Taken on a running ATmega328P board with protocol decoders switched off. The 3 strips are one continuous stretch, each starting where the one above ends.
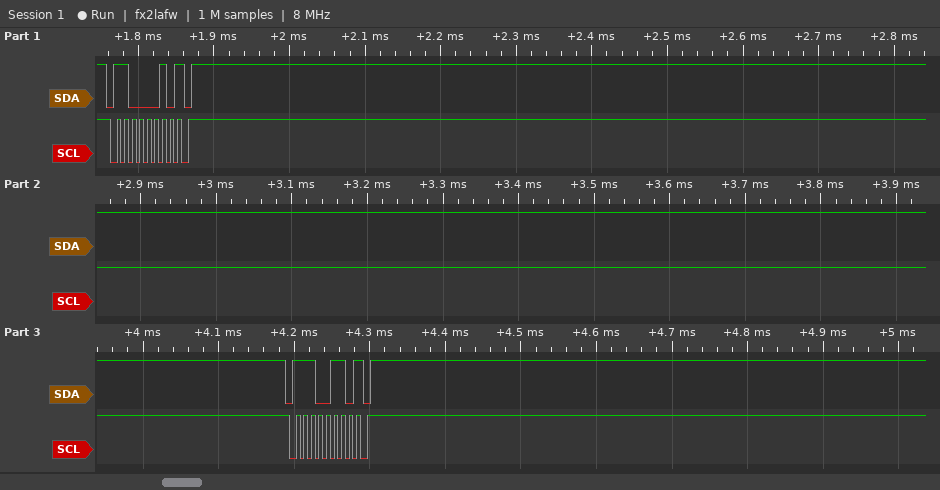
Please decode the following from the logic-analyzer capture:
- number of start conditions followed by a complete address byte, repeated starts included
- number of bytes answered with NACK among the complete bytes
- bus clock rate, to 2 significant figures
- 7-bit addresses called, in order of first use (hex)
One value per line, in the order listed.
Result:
2
2
100 kHz
0x61 0x73
